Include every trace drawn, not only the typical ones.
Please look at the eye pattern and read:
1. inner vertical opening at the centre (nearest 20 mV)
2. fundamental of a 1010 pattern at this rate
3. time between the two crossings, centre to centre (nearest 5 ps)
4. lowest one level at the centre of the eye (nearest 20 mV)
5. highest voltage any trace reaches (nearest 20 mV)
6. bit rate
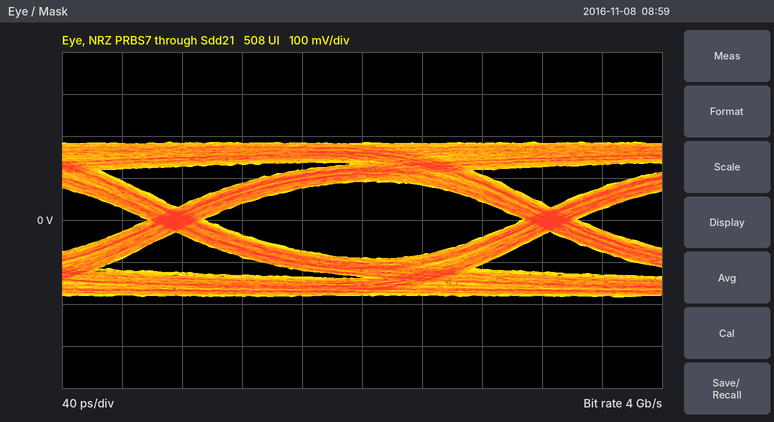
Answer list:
180 mV
2 GHz
250 ps
100 mV
180 mV
4 Gb/s
